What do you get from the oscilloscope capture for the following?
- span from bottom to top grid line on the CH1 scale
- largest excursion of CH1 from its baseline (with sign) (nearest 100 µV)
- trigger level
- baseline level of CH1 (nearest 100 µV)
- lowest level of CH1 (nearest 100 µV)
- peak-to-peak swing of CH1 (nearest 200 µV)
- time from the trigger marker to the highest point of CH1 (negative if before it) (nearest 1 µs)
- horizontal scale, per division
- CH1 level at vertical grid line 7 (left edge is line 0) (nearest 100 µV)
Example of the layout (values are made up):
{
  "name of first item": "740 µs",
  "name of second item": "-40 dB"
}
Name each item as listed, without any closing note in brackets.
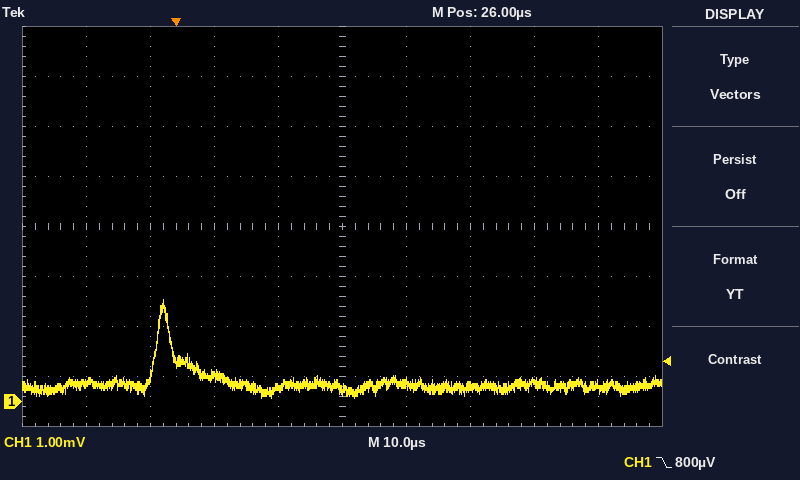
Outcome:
{
  "span from bottom to top grid line on the CH1 scale": "8 mV",
  "largest excursion of CH1 from its baseline (with sign)": "+1.7 mV",
  "trigger level": "800 µV",
  "baseline level of CH1": "300 µV",
  "lowest level of CH1": "100 µV",
  "peak-to-peak swing of CH1": "2.0 mV",
  "time from the trigger marker to the highest point of CH1 (negative if before it)": "-2 µs",
  "horizontal scale, per division": "10 µs",
  "CH1 level at vertical grid line 7 (left edge is line 0)": "300 µV"
}
